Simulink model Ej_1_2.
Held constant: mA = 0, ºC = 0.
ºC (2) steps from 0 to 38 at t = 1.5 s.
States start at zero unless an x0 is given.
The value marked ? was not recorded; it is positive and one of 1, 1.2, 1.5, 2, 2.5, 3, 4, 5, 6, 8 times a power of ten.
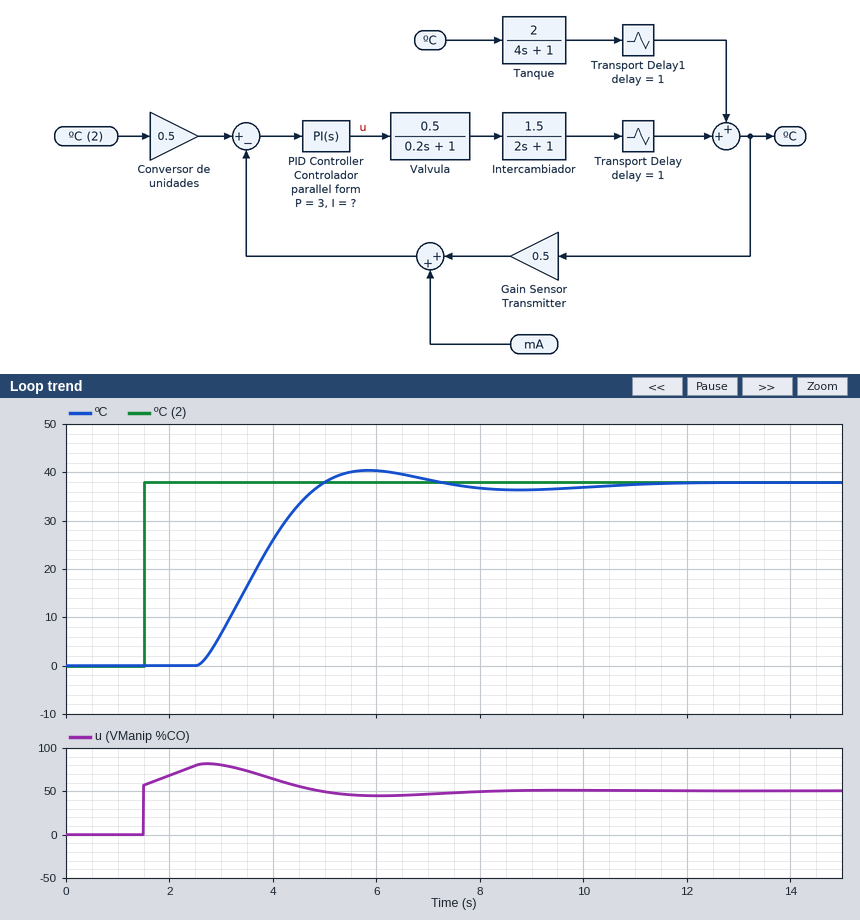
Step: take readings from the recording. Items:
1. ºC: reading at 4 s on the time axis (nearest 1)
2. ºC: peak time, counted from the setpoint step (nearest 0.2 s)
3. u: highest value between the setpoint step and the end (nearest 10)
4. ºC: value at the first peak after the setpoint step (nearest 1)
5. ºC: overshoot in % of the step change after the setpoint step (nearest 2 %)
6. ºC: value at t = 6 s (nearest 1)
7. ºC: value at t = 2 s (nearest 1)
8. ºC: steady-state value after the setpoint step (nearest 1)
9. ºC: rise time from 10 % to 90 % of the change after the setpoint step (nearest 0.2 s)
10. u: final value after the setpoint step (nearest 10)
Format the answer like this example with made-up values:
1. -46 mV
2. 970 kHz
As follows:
1. 26
2. 4.4 s
3. 80
4. 40
5. 6 %
6. 40
7. 0
8. 38
9. 1.8 s
10. 50
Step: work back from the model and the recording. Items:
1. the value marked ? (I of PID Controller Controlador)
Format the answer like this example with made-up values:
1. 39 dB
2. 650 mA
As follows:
1. 1.2
